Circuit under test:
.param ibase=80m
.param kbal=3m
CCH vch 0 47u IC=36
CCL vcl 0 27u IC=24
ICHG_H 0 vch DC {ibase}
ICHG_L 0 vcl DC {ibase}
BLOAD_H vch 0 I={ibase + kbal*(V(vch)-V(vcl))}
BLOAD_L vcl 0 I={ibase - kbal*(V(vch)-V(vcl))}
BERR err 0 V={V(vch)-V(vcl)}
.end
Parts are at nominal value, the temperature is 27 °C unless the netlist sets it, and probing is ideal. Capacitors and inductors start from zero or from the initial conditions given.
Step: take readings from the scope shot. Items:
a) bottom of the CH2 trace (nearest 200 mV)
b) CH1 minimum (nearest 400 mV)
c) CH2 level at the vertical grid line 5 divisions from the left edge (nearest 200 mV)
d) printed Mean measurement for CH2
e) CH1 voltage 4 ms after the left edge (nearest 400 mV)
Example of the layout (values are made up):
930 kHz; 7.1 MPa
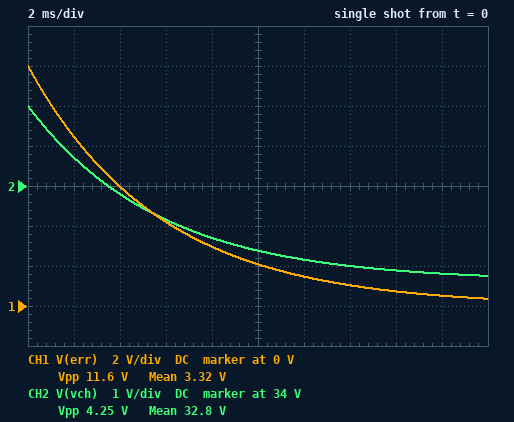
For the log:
31.8 V; 400 mV; 32.4 V; 32.8 V; 6.0 V
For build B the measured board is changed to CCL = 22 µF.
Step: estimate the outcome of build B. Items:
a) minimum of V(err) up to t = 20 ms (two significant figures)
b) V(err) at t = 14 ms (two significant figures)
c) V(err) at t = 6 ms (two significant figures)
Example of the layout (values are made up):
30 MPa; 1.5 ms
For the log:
220 mV; 730 mV; 3.6 V
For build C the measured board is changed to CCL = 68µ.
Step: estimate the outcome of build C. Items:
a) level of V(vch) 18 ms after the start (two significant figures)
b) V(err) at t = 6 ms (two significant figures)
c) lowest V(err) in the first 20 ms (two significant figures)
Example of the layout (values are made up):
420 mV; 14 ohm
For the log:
30 V; 6.3 V; 1.4 V
